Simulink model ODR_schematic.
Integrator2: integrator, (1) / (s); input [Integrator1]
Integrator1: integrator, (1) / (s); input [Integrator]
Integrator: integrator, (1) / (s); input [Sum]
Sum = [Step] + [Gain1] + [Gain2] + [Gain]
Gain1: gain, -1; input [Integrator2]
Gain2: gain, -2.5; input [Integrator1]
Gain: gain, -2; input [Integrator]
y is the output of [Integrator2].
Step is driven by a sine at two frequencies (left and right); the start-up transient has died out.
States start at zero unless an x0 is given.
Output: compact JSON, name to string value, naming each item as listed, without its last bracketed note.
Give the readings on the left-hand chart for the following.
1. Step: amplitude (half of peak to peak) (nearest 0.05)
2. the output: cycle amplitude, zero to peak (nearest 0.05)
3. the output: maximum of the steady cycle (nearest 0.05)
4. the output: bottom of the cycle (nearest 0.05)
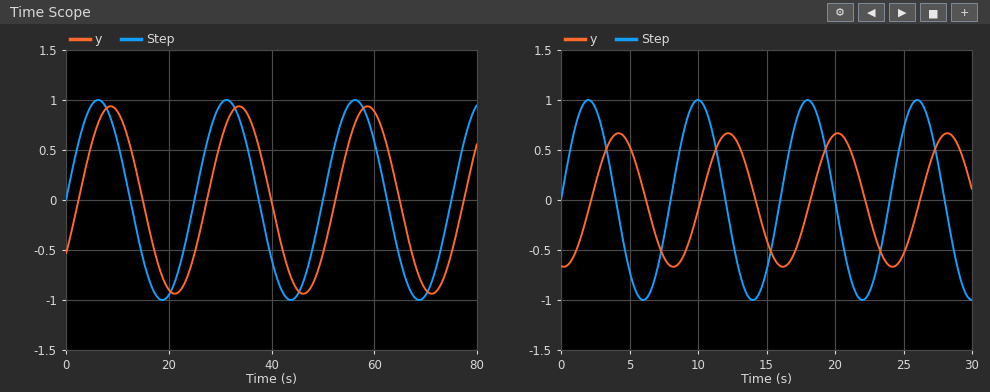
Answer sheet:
{"Step: amplitude (half of peak to peak)": "1.00", "the output: cycle amplitude, zero to peak": "0.95", "the output: maximum of the steady cycle": "0.95", "the output: bottom of the cycle": "-0.95"}
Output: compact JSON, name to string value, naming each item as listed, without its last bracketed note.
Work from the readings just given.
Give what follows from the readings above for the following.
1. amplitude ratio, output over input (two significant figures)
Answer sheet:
{"amplitude ratio, output over input": "0.95"}
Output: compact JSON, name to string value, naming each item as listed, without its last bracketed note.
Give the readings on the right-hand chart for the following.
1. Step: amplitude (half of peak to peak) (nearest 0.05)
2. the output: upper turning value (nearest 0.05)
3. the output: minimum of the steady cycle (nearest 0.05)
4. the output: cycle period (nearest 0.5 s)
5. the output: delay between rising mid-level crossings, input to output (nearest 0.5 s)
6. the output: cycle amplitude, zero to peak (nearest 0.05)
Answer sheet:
{"Step: amplitude (half of peak to peak)": "1.00", "the output: upper turning value": "0.65", "the output: minimum of the steady cycle": "-0.65", "the output: cycle period": "8.0 s", "the output: delay between rising mid-level crossings, input to output": "2.0 s", "the output: cycle amplitude, zero to peak": "0.65"}
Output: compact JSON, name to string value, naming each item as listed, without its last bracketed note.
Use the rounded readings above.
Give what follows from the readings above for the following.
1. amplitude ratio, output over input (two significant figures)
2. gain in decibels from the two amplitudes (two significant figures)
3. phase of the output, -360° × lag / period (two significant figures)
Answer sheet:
{"amplitude ratio, output over input": "0.65", "gain in decibels from the two amplitudes": "-3.7 dB", "phase of the output, -360° × lag / period": "-90°"}
